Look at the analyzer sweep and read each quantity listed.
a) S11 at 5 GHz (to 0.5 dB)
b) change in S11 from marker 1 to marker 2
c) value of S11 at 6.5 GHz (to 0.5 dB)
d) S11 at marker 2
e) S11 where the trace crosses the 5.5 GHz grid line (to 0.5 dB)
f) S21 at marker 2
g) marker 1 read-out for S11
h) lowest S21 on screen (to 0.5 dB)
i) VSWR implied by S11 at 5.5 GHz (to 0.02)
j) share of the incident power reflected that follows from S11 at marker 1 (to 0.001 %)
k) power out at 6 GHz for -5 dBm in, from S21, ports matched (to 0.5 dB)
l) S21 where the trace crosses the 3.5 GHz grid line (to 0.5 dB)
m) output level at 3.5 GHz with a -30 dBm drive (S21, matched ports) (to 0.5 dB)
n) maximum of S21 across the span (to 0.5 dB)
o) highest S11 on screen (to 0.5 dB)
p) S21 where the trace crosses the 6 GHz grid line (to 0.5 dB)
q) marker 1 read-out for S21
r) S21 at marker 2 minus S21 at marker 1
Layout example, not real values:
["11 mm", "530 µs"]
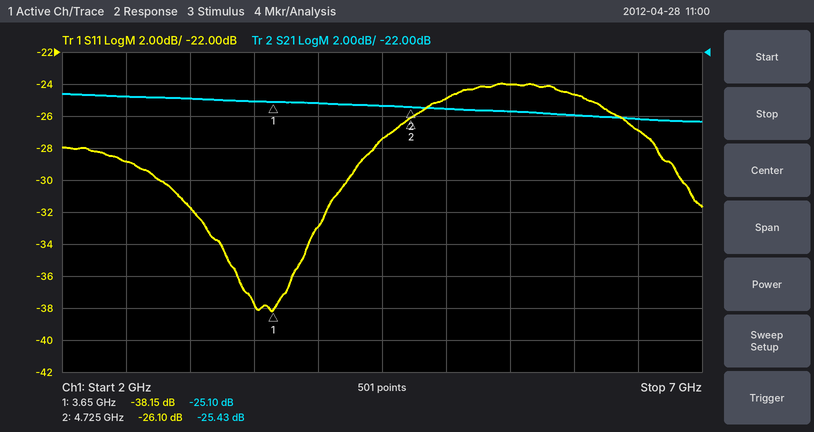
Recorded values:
["-25.0 dB", "12.05 dB", "-27.0 dB", "-26.10 dB", "-24.0 dB", "-25.43 dB", "-38.15 dB", "-26.5 dB", "1.14", "0.015 %", "-31.0 dBm", "-25.0 dB", "-55.0 dBm", "-24.5 dB", "-24.0 dB", "-26.0 dB", "-25.10 dB", "-0.33 dB"]
